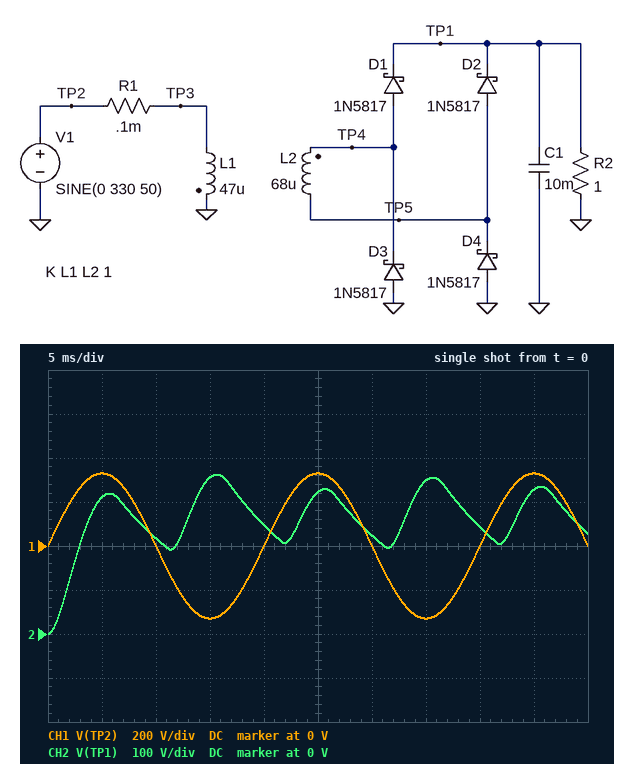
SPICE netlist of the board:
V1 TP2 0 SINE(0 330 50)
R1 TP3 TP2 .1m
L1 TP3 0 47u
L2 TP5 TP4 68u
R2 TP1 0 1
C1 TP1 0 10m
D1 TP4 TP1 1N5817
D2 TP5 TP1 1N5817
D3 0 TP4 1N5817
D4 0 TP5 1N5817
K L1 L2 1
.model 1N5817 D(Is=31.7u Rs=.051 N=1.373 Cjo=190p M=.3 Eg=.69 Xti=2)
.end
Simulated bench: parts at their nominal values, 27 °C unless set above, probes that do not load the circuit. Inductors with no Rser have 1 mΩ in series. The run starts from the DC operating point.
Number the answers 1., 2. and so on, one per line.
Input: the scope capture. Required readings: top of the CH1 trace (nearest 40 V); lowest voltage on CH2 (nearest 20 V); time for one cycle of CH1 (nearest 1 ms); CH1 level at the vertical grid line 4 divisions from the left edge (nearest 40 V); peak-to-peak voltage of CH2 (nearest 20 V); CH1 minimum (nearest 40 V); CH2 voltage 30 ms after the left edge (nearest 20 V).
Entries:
1. 320 V
2. 0 V
3. 20 ms
4. 0 V
5. 360 V
6. -320 V
7. 220 V
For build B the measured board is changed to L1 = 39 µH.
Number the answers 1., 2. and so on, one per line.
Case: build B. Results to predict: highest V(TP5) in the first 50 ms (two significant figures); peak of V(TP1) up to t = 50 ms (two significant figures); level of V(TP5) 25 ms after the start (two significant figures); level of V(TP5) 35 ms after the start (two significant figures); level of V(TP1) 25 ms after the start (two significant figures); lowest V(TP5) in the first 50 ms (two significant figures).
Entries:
1. 390 V
2. 400 V
3. 380 V
4. -31 V
5. 350 V
6. -50 V
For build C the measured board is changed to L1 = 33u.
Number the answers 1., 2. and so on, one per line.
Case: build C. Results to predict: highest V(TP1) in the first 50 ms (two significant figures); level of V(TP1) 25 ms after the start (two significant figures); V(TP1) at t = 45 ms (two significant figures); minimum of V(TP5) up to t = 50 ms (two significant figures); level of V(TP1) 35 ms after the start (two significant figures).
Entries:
1. 440 V
2. 380 V
3. 390 V
4. -55 V
5. 420 V
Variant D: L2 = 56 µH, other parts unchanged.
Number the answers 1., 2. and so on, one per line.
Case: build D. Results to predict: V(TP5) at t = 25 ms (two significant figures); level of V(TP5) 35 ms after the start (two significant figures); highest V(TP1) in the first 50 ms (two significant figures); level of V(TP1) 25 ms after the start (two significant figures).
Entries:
1. 320 V
2. -26 V
3. 330 V
4. 290 V
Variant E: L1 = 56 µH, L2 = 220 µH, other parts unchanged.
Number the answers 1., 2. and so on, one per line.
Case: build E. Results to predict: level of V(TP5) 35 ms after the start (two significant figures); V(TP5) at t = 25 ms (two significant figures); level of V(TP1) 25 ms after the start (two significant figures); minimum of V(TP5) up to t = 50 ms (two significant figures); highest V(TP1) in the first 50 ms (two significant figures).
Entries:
1. -48 V
2. 580 V
3. 530 V
4. -74 V
5. 590 V
